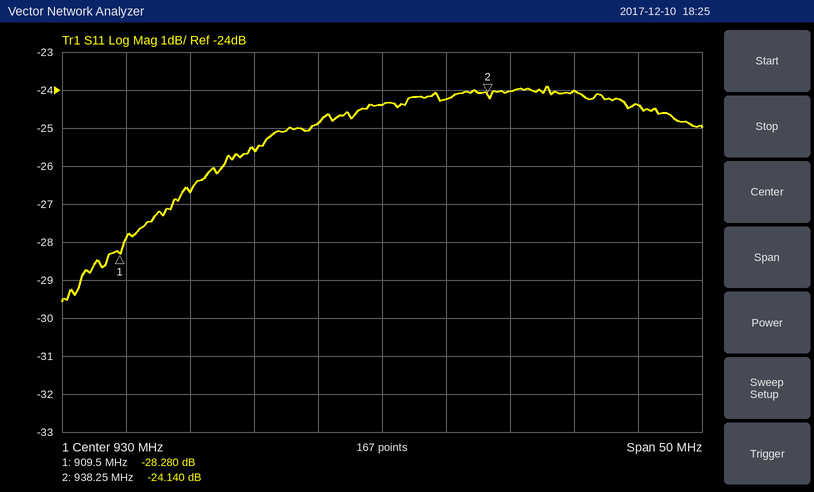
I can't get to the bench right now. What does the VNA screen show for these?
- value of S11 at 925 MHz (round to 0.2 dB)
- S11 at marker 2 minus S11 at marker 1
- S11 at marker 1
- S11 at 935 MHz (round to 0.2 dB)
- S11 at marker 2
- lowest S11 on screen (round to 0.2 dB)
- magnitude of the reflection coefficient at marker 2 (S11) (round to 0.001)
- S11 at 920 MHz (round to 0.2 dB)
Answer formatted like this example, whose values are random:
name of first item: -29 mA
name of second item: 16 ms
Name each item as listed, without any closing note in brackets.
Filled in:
value of S11 at 925 MHz: -24.8 dB
S11 at marker 2 minus S11 at marker 1: 4.140 dB
S11 at marker 1: -28.280 dB
S11 at 935 MHz: -24.2 dB
S11 at marker 2: -24.140 dB
lowest S11 on screen: -29.6 dB
magnitude of the reflection coefficient at marker 2 (S11): 0.062
S11 at 920 MHz: -25.6 dB
